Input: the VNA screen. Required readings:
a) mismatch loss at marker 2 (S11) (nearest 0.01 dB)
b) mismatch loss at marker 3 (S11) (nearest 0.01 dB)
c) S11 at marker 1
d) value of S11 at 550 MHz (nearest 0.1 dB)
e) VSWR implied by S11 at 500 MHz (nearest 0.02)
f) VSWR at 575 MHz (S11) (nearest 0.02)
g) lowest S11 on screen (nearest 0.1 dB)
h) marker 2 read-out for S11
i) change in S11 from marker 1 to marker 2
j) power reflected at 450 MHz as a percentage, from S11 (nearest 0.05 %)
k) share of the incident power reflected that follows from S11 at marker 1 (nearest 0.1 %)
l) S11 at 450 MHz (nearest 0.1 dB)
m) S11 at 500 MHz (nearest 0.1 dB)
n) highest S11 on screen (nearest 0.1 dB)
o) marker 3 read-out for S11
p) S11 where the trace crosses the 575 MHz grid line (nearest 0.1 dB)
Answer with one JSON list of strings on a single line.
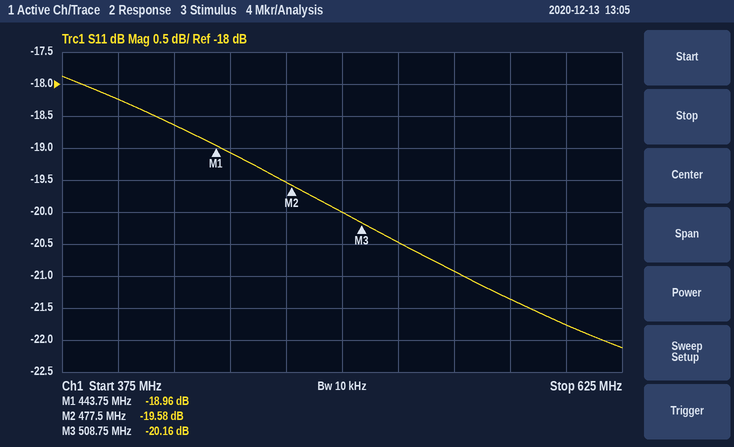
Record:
["0.05 dB", "0.04 dB", "-18.96 dB", "-20.9 dB", "1.22", "1.18", "-22.1 dB", "-19.58 dB", "-0.62 dB", "1.25 %", "1.3 %", "-19.1 dB", "-20.0 dB", "-17.9 dB", "-20.16 dB", "-21.4 dB"]
